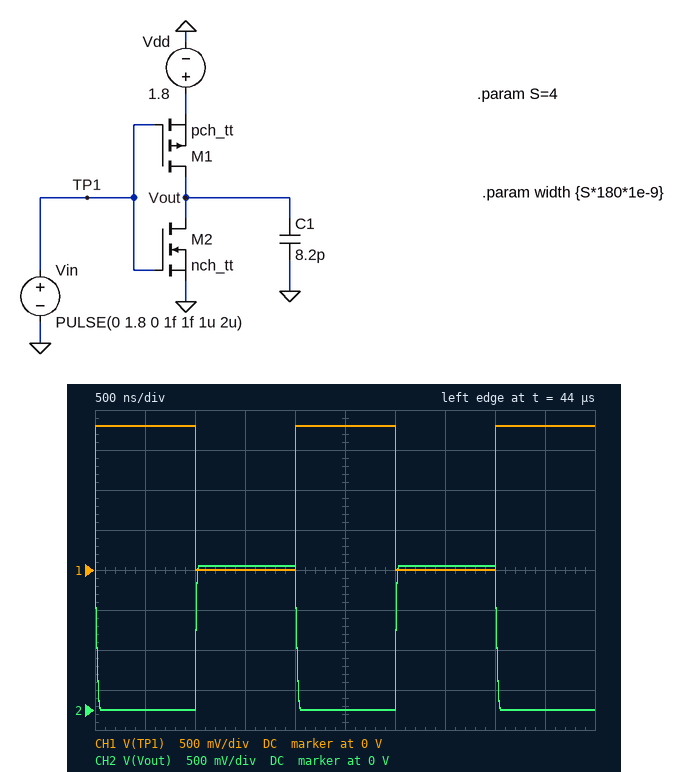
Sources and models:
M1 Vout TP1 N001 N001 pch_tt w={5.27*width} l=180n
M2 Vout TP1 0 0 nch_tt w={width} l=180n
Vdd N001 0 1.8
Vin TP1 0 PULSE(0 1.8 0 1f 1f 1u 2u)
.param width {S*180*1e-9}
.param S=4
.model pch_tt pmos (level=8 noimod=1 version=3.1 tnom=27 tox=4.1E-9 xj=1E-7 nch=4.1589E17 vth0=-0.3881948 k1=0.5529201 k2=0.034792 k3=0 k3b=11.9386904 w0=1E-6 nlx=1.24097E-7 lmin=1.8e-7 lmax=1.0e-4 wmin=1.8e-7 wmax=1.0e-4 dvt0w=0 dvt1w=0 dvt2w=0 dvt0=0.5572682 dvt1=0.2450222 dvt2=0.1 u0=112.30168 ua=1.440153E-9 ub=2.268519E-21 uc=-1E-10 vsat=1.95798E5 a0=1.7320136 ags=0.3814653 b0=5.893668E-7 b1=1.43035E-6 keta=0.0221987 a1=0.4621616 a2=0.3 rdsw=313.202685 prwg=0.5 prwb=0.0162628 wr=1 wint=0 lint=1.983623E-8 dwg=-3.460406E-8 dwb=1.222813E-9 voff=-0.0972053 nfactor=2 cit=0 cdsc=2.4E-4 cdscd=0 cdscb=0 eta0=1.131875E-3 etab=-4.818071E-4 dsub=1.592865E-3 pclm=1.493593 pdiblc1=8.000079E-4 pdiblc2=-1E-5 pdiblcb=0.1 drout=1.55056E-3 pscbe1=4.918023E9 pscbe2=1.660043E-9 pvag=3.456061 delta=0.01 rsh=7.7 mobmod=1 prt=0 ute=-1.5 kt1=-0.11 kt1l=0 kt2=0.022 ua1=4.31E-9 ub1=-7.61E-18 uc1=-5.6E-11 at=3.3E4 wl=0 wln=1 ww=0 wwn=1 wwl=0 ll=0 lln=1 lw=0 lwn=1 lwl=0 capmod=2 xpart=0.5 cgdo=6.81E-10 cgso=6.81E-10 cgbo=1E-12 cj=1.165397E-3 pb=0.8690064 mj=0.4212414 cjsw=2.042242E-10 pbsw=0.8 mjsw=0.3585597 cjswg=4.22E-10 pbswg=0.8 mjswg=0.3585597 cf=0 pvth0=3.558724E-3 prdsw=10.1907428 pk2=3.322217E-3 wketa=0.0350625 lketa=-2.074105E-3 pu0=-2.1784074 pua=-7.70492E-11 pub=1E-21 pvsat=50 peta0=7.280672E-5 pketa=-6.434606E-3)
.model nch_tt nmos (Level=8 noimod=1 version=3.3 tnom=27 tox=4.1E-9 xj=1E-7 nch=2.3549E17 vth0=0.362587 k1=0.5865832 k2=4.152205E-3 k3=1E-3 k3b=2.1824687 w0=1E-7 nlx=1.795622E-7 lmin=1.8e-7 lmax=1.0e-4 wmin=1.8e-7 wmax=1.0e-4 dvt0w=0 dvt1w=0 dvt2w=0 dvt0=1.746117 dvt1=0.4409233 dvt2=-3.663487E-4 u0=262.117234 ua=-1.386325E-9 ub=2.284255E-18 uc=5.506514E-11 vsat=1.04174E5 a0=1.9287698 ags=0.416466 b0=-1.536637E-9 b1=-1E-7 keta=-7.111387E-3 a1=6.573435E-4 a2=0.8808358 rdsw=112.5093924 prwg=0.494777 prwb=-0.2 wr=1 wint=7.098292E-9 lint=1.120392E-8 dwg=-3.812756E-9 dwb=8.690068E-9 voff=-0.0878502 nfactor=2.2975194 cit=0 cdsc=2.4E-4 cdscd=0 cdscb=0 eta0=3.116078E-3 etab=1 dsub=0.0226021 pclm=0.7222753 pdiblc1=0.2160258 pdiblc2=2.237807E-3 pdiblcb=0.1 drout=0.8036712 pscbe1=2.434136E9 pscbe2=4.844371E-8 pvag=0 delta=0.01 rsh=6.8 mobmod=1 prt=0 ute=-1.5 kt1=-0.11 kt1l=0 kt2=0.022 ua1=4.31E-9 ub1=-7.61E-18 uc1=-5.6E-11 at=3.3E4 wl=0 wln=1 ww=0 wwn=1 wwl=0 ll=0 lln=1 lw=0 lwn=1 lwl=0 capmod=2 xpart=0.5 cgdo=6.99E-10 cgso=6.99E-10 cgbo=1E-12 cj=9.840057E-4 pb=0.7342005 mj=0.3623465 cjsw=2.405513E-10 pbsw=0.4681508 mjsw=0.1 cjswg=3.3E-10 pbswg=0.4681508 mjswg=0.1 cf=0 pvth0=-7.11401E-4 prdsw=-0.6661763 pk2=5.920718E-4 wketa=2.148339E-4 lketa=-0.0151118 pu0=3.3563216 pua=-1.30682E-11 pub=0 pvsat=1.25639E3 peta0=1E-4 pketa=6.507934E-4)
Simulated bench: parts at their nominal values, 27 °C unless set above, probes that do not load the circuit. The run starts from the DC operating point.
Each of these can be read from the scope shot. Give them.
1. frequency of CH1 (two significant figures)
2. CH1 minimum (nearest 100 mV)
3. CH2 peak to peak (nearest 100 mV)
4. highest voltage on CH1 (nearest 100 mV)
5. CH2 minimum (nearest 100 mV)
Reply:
500 kHz
0 V
1.8 V
1.8 V
0 V
